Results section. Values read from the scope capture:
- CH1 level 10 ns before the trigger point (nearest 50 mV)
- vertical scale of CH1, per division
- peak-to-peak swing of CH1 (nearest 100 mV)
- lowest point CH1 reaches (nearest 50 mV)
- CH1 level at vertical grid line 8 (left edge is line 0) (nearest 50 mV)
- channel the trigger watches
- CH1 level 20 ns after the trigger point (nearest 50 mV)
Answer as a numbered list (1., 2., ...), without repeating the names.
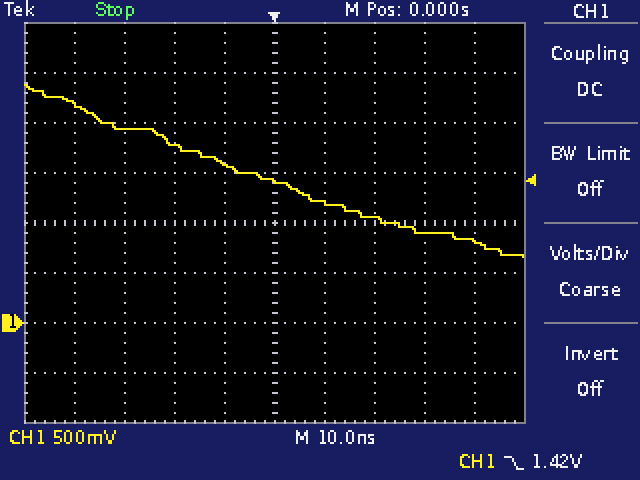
1. 1.60 V
2. 500 mV
3. 1.70 V
4. 650 mV
5. 900 mV
6. CH1
7. 1.05 V
